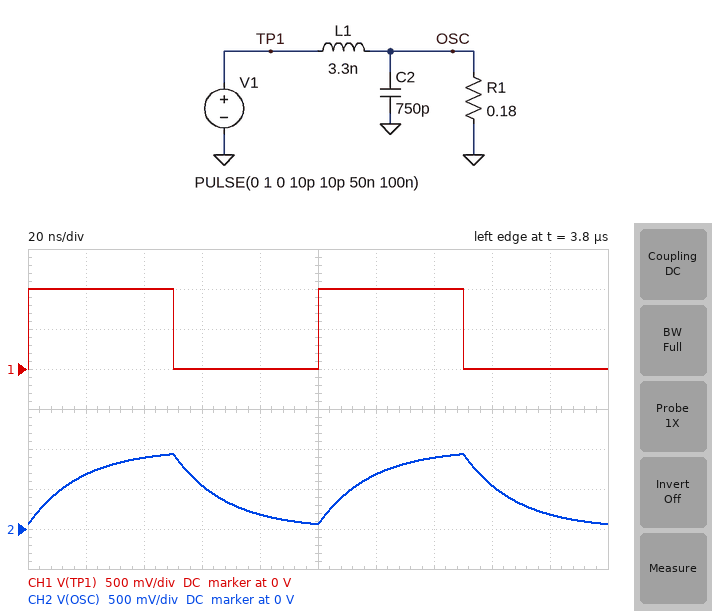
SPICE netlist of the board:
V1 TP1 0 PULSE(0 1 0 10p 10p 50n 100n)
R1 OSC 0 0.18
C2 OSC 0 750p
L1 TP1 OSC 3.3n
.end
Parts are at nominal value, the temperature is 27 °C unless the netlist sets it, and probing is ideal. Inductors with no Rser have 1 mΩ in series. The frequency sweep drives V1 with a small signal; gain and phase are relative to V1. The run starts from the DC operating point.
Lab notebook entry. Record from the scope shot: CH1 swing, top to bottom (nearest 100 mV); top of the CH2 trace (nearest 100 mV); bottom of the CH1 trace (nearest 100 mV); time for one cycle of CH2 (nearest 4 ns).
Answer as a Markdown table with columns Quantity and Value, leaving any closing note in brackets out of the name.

| Quantity | Value |
|---|---|
| CH1 swing, top to bottom | 1.0 V |
| top of the CH2 trace | 900 mV |
| bottom of the CH1 trace | 0 V |
| time for one cycle of CH2 | 100 ns |
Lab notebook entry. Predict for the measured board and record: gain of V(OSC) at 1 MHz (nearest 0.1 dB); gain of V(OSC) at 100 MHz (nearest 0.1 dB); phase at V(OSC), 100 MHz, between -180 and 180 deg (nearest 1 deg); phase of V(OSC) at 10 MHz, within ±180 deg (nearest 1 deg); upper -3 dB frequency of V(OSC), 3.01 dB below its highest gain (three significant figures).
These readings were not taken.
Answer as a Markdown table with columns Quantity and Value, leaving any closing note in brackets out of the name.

| Quantity | Value |
|---|---|
| gain of V(OSC) at 1 MHz | -0.1 dB |
| gain of V(OSC) at 100 MHz | -21.2 dB |
| phase at V(OSC), 100 MHz, between -180 and 180 deg | -90 deg |
| phase of V(OSC) at 10 MHz, within ±180 deg | -49 deg |
| upper -3 dB frequency of V(OSC), 3.01 dB below its highest gain | 8.79 MHz |
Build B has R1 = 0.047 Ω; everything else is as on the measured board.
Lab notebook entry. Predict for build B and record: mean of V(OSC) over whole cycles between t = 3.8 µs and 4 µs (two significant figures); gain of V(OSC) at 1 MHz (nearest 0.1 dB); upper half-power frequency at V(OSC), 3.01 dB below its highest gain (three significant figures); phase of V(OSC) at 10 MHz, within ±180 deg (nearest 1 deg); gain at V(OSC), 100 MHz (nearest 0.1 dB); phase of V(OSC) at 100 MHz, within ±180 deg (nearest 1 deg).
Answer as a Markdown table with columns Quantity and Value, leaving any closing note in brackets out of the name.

| Quantity | Value |
|---|---|
| mean of V(OSC) over whole cycles between t = 3.8 µs and 4 µs | 490 mV |
| gain of V(OSC) at 1 MHz | -0.9 dB |
| upper half-power frequency at V(OSC), 3.01 dB below its highest gain | 2.32 MHz |
| phase of V(OSC) at 10 MHz, within ±180 deg | -77 deg |
| gain at V(OSC), 100 MHz | -32.9 dB |
| phase of V(OSC) at 100 MHz, within ±180 deg | -90 deg |
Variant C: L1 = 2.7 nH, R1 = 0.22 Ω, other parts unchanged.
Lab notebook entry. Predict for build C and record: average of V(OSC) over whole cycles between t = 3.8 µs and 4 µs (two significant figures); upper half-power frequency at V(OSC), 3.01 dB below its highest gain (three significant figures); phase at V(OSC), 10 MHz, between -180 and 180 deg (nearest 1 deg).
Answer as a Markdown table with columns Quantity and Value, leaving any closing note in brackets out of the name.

| Quantity | Value |
|---|---|
| average of V(OSC) over whole cycles between t = 3.8 µs and 4 µs | 500 mV |
| upper half-power frequency at V(OSC), 3.01 dB below its highest gain | 13.2 MHz |
| phase at V(OSC), 10 MHz, between -180 and 180 deg | -38 deg |
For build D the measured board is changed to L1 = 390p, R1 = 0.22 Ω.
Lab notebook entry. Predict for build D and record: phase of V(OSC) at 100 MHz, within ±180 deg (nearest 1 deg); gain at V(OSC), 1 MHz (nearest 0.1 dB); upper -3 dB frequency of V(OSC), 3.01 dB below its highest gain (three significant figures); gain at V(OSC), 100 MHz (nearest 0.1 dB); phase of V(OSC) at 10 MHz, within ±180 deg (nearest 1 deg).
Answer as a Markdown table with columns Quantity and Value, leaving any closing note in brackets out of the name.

| Quantity | Value |
|---|---|
| phase of V(OSC) at 100 MHz, within ±180 deg | -51 deg |
| gain at V(OSC), 1 MHz | 0 dB |
| upper -3 dB frequency of V(OSC), 3.01 dB below its highest gain | 99.3 MHz |
| gain at V(OSC), 100 MHz | -3.1 dB |
| phase of V(OSC) at 10 MHz, within ±180 deg | -6 deg |
